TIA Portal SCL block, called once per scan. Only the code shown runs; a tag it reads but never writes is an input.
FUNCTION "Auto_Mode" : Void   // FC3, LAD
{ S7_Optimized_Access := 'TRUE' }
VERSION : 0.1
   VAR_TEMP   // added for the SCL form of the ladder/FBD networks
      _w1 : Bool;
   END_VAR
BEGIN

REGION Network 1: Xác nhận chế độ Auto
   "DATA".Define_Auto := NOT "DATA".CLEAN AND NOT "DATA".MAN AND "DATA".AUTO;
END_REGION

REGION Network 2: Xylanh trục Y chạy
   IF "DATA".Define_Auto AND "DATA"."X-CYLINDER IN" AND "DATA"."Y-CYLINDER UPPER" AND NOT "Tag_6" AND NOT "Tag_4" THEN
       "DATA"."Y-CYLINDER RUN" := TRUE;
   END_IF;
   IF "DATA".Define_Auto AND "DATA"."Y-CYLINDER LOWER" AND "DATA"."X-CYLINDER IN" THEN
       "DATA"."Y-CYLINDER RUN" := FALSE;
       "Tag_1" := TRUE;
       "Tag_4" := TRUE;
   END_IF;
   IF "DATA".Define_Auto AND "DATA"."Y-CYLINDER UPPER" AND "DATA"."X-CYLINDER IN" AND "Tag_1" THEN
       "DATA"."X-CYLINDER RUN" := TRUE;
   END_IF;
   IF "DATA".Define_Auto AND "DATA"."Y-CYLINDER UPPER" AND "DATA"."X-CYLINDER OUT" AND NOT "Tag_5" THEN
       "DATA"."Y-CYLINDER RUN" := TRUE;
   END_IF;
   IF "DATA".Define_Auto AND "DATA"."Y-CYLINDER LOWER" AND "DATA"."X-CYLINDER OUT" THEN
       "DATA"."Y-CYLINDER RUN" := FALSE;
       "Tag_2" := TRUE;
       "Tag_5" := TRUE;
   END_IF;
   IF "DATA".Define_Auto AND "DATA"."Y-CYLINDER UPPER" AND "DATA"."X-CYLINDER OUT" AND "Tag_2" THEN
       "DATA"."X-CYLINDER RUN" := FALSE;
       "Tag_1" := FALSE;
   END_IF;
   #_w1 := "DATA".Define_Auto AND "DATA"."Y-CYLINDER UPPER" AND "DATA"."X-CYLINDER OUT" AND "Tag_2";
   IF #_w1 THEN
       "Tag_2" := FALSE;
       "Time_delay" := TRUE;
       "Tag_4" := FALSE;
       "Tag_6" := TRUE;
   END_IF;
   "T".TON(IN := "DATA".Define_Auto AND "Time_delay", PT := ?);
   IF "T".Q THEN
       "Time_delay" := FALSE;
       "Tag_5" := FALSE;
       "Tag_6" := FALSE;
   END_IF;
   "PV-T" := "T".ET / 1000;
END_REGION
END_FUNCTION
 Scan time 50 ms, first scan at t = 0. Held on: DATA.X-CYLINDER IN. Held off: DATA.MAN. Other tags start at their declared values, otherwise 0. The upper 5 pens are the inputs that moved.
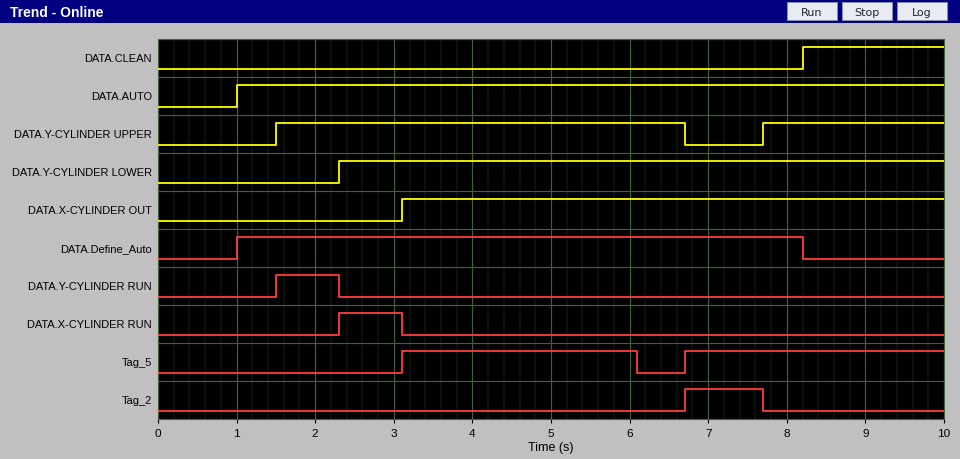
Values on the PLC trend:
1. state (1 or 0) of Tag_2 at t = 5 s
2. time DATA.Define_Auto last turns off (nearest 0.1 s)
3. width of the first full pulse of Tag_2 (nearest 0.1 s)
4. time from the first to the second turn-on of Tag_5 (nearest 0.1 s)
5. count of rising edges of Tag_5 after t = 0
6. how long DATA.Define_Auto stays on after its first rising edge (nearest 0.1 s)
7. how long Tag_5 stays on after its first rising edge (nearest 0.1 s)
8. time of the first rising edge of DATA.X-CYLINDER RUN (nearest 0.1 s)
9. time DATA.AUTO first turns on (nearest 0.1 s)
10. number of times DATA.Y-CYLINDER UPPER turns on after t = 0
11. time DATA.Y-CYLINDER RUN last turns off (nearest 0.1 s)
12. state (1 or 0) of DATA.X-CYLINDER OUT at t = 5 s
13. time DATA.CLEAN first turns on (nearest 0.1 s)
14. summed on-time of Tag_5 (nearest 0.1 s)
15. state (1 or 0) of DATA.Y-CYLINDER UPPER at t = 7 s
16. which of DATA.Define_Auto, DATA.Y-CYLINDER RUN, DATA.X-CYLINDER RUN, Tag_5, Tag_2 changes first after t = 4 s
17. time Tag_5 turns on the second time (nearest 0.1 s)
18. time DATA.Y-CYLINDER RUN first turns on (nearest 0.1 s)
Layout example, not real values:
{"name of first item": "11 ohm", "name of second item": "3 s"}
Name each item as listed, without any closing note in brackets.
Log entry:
{"state (1 or 0) of Tag_2 at t = 5 s": "0", "time DATA.Define_Auto last turns off": "8.2 s", "width of the first full pulse of Tag_2": "1.0 s", "time from the first to the second turn-on of Tag_5": "3.6 s", "count of rising edges of Tag_5 after t = 0": "2", "how long DATA.Define_Auto stays on after its first rising edge": "7.2 s", "how long Tag_5 stays on after its first rising edge": "3.0 s", "time of the first rising edge of DATA.X-CYLINDER RUN": "2.3 s", "time DATA.AUTO first turns on": "1.0 s", "number of times DATA.Y-CYLINDER UPPER turns on after t = 0": "2", "time DATA.Y-CYLINDER RUN last turns off": "2.3 s", "state (1 or 0) of DATA.X-CYLINDER OUT at t = 5 s": "1", "time DATA.CLEAN first turns on": "8.2 s", "summed on-time of Tag_5": "6.3 s", "state (1 or 0) of DATA.Y-CYLINDER UPPER at t = 7 s": "0", "which of DATA.Define_Auto, DATA.Y-CYLINDER RUN, DATA.X-CYLINDER RUN, Tag_5, Tag_2 changes first after t = 4 s": "Tag_5", "time Tag_5 turns on the second time": "6.7 s", "time DATA.Y-CYLINDER RUN first turns on": "1.5 s"}
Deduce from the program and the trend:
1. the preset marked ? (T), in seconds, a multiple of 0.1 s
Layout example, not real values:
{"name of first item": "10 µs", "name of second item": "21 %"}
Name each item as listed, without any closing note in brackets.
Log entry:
{"the preset marked ? (T), in seconds, a multiple of 0.1 s": "3.0 s"}
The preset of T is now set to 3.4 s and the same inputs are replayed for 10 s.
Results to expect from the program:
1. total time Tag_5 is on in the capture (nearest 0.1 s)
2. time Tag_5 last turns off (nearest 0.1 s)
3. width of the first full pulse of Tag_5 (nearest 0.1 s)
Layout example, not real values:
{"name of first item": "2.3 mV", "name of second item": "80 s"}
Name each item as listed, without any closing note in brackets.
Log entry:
{"total time Tag_5 is on in the capture": "6.7 s", "time Tag_5 last turns off": "6.5 s", "width of the first full pulse of Tag_5": "3.4 s"}
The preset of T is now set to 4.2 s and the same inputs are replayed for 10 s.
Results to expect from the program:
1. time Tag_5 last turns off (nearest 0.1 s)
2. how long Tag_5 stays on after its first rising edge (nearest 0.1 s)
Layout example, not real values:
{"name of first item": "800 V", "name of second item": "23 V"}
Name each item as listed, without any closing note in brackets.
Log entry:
{"time Tag_5 last turns off": "7.3 s", "how long Tag_5 stays on after its first rising edge": "4.2 s"}
